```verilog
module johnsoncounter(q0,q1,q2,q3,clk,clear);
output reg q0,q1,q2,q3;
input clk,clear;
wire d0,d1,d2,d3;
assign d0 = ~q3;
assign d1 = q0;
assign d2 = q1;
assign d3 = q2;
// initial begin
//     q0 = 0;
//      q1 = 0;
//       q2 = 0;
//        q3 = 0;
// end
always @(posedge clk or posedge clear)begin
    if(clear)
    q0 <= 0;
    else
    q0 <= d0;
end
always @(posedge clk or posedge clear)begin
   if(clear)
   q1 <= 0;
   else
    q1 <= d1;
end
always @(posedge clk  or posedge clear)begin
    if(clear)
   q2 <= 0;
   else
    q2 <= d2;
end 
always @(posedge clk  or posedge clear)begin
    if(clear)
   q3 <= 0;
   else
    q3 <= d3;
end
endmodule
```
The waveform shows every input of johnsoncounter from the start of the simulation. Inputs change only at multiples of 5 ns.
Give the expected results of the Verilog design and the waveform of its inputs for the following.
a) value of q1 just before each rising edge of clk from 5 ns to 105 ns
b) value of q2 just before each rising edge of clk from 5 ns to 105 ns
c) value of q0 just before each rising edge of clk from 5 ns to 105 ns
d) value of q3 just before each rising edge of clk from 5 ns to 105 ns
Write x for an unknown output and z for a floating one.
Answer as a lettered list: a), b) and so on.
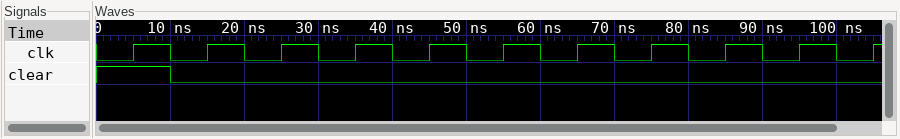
a) 0 0 0 1 1 1 1 0 0 0 0
b) 0 0 0 0 1 1 1 1 0 0 0
c) 0 0 1 1 1 1 0 0 0 0 1
d) 0 0 0 0 0 1 1 1 1 0 0
